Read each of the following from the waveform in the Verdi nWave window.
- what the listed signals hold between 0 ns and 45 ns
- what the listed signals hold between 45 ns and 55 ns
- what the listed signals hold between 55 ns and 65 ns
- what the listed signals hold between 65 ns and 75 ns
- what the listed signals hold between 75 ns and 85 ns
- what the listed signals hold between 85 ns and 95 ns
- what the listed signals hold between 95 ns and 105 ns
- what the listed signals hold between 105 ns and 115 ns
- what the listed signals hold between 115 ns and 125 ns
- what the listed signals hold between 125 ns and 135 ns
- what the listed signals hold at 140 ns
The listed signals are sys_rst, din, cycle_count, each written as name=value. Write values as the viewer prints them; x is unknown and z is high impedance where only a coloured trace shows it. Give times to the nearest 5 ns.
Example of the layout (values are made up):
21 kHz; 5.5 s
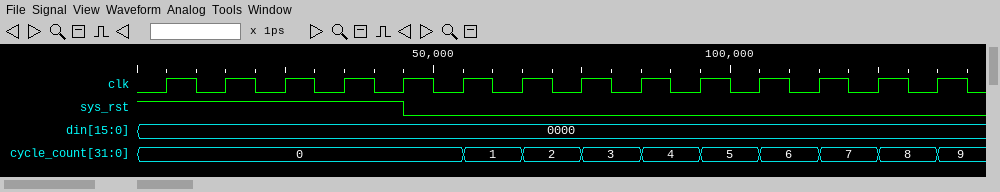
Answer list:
sys_rst=1, din=0000, cycle_count=0; sys_rst=0, din=0000, cycle_count=0; sys_rst=0, din=0000, cycle_count=1; sys_rst=0, din=0000, cycle_count=2; sys_rst=0, din=0000, cycle_count=3; sys_rst=0, din=0000, cycle_count=4; sys_rst=0, din=0000, cycle_count=5; sys_rst=0, din=0000, cycle_count=6; sys_rst=0, din=0000, cycle_count=7; sys_rst=0, din=0000, cycle_count=8; sys_rst=0, din=0000, cycle_count=9
